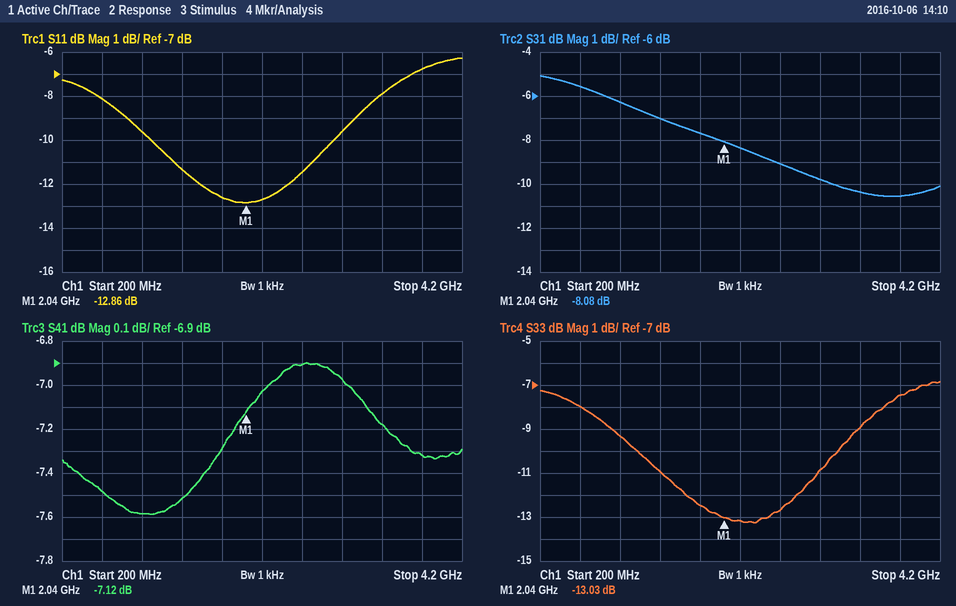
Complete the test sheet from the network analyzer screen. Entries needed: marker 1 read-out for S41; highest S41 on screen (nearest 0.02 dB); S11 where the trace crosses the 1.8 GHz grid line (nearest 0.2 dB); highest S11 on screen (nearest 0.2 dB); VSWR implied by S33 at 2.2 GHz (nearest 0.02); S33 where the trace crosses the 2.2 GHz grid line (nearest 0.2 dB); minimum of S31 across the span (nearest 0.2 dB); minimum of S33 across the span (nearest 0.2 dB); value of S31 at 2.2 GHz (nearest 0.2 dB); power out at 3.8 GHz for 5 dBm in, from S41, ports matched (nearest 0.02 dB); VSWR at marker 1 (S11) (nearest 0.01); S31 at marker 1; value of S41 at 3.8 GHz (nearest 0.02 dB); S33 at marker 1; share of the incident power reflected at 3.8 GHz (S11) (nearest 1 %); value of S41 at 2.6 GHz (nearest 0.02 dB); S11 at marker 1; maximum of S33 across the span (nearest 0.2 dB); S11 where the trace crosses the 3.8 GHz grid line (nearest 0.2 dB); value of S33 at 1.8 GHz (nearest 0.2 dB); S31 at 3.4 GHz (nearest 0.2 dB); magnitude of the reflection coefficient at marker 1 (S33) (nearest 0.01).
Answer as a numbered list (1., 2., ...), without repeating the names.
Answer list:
1. -7.12 dB
2. -6.90 dB
3. -12.6 dB
4. -6.2 dB
5. 1.56
6. -13.2 dB
7. -10.6 dB
8. -13.2 dB
9. -8.4 dB
10. -2.32 dBm
11. 1.59
12. -8.08 dB
13. -7.32 dB
14. -13.03 dB
15. 21 %
16. -6.90 dB
17. -12.86 dB
18. -6.8 dB
19. -6.8 dB
20. -12.4 dB
21. -10.4 dB
22. 0.22
